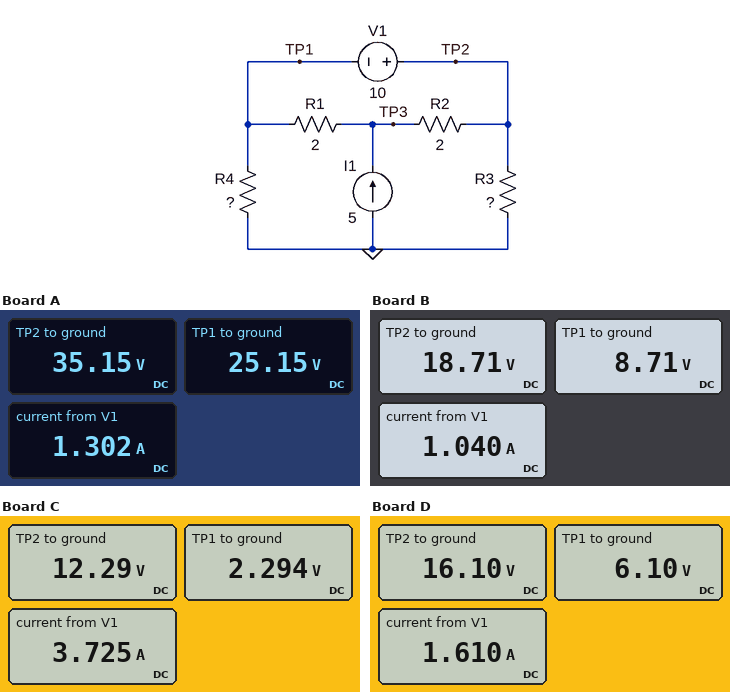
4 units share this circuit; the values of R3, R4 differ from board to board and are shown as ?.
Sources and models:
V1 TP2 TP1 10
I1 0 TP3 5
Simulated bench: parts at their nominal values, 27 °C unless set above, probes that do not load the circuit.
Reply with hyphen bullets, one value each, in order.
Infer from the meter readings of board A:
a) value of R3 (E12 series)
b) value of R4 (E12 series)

- 27 Ω
- 6.8 Ω
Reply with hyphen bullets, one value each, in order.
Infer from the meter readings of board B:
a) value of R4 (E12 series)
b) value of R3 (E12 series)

- 2.2 Ω
- 18 Ω
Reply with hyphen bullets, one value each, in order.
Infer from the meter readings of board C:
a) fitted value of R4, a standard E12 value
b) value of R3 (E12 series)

- 1.8 Ω
- 3.3 Ω
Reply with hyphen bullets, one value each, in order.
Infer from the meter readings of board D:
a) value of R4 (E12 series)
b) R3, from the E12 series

- 1.8 Ω
- 10 Ω
